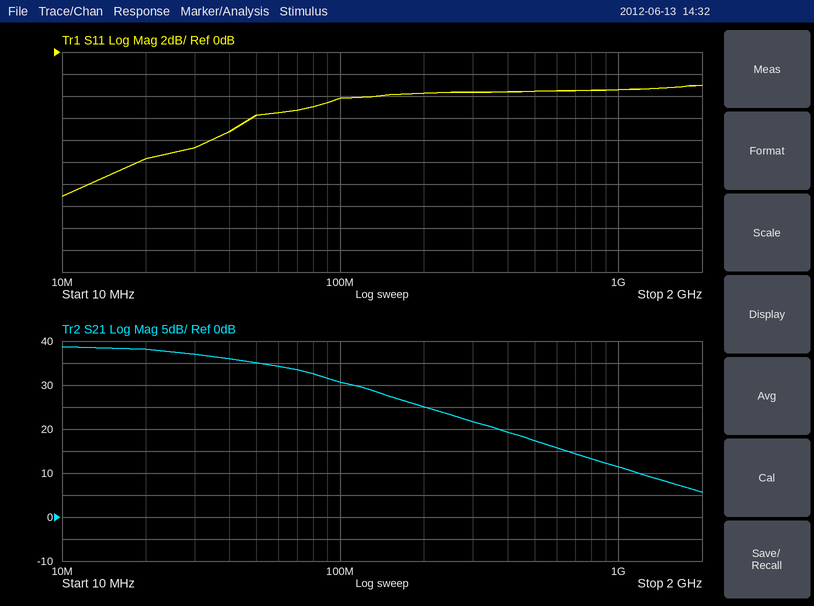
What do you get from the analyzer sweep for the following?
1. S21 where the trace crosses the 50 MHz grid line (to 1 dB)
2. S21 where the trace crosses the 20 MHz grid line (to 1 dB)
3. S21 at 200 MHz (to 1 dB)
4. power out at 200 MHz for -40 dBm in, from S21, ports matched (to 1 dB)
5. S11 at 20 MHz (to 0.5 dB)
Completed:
35 dB
38 dB
25 dB
-15 dBm
-9.5 dB
